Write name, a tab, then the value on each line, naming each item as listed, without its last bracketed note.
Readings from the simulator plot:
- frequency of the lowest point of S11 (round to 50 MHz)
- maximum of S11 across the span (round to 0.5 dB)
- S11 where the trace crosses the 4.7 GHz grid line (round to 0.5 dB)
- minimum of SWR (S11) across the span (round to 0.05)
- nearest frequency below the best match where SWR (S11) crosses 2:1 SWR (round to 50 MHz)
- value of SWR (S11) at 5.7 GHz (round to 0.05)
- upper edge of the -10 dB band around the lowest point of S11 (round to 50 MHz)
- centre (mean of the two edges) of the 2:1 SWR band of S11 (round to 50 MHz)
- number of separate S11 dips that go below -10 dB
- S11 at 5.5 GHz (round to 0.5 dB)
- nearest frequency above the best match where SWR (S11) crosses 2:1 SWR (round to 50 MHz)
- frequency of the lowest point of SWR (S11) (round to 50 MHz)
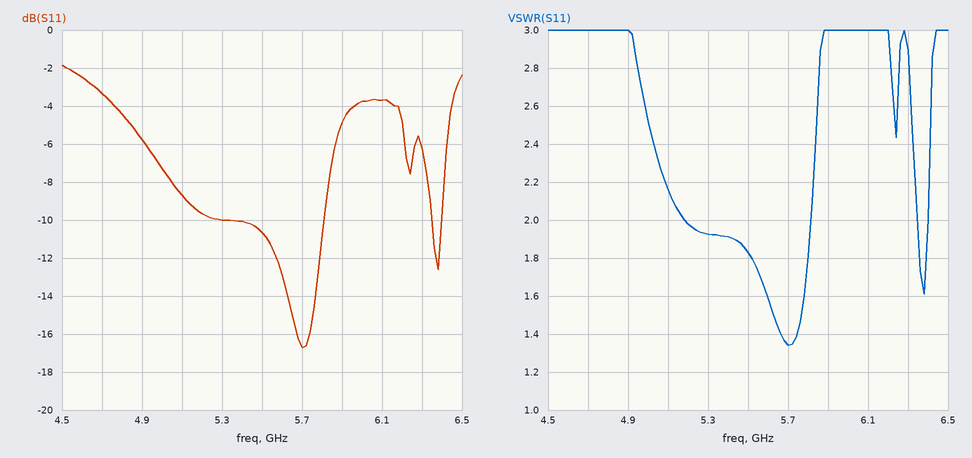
frequency of the lowest point of S11	5.70 GHz
maximum of S11 across the span	-2.0 dB
S11 where the trace crosses the 4.7 GHz grid line	-3.5 dB
minimum of SWR (S11) across the span	1.35
nearest frequency below the best match where SWR (S11) crosses 2:1 SWR	5.20 GHz
value of SWR (S11) at 5.7 GHz	1.35
upper edge of the -10 dB band around the lowest point of S11	5.80 GHz
centre (mean of the two edges) of the 2:1 SWR band of S11	5.50 GHz
number of separate S11 dips that go below -10 dB	2
S11 at 5.5 GHz	-10.5 dB
nearest frequency above the best match where SWR (S11) crosses 2:1 SWR	5.80 GHz
frequency of the lowest point of SWR (S11)	5.70 GHz
